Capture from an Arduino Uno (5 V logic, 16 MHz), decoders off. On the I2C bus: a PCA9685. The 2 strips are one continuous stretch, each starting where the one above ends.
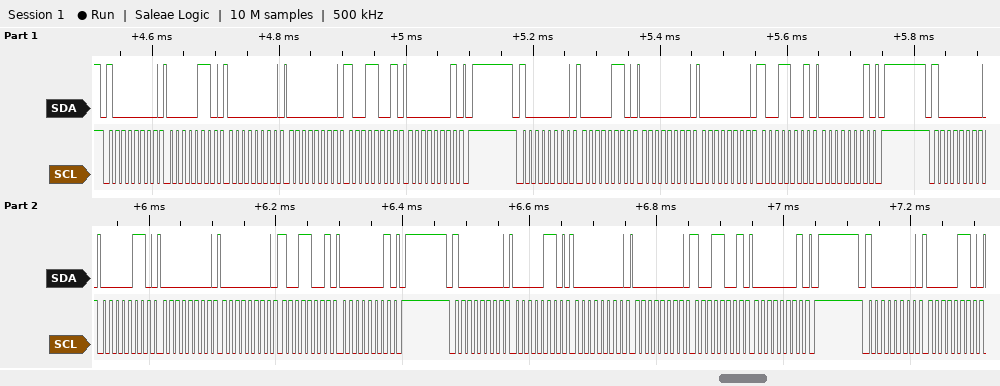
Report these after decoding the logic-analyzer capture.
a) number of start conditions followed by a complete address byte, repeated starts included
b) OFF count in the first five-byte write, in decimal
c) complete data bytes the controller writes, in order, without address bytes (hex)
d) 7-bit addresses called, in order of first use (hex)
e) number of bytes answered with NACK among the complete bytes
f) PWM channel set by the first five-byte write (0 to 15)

5
409
06 00 00 99 01 06 00 00 99 01 06 00 00 99 01 06 00 00 99 01 06
0x40
0
0
